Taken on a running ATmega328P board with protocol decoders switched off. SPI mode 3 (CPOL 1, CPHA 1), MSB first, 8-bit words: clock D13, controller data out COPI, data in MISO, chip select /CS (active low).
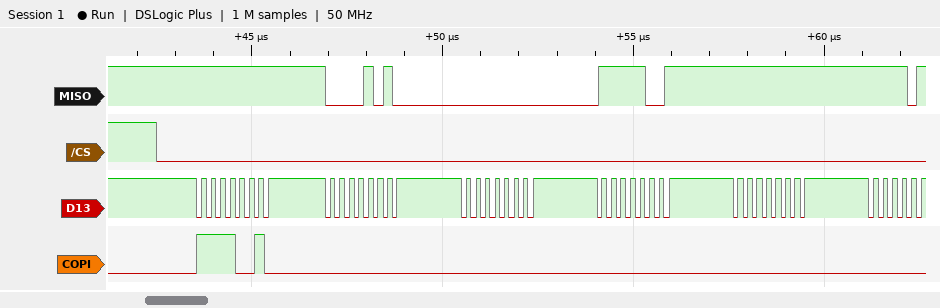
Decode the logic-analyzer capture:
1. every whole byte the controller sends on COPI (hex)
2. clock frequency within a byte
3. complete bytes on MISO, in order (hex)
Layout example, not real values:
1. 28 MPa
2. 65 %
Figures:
1. F2 00 00 00 00
2. 4 MHz
3. FF 0A 00 F9 FF
